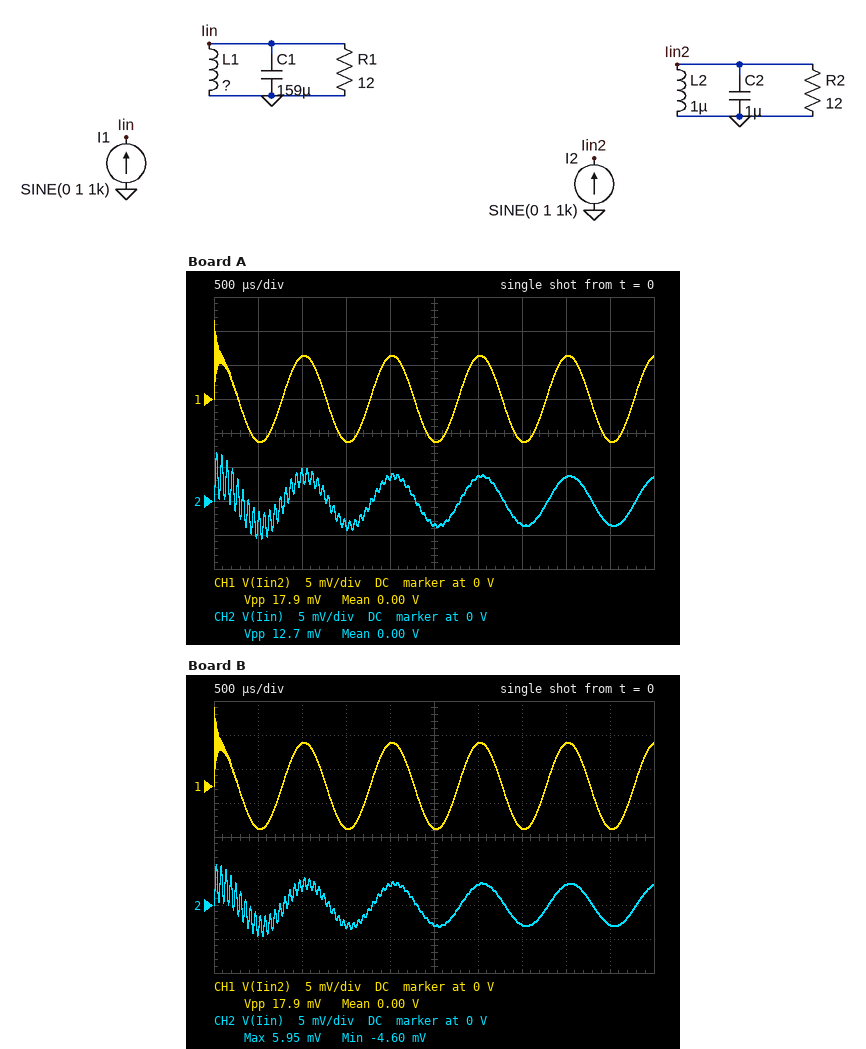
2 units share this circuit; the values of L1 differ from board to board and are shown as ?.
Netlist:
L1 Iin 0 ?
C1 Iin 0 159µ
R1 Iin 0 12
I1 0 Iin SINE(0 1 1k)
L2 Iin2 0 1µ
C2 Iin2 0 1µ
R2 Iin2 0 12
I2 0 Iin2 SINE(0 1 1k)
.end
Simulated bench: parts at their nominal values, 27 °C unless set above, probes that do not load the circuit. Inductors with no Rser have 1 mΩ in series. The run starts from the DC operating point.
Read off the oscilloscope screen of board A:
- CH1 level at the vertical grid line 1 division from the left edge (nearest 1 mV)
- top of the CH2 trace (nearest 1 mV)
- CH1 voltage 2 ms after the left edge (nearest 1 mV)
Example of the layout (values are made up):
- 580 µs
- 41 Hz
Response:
- -6 mV
- 7 mV
- 6 mV
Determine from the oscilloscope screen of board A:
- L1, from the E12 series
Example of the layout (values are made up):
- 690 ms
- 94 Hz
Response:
- 560 nH
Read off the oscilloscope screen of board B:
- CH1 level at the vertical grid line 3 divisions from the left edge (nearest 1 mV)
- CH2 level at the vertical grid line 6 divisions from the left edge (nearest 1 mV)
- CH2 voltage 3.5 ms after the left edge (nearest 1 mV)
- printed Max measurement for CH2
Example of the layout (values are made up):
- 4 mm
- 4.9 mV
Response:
- -6 mV
- 3 mV
- -3 mV
- 5.95 mV
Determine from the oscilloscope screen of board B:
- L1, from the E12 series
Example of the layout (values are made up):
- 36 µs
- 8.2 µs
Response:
- 470 nH
